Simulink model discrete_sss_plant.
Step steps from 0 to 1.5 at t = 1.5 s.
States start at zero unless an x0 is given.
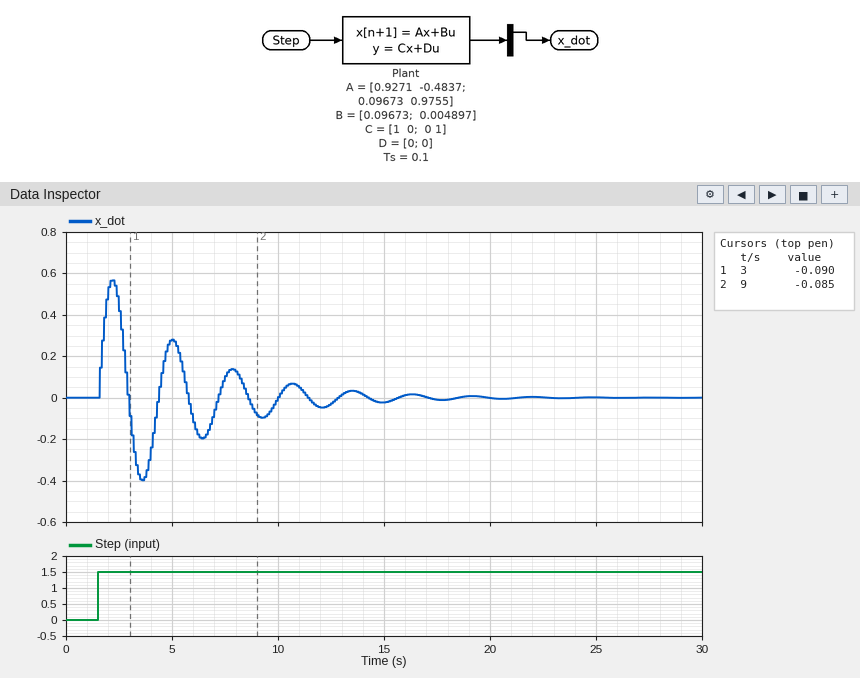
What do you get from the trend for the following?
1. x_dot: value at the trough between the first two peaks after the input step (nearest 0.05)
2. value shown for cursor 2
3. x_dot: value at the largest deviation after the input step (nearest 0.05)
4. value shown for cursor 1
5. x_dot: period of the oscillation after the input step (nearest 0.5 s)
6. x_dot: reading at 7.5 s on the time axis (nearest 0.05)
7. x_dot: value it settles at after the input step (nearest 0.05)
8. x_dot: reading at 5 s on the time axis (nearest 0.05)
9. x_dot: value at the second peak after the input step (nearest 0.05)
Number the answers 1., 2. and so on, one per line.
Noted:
1. -0.40
2. -0.085
3. 0.55
4. -0.090
5. 3.0 s
6. 0.10
7. 0.00
8. 0.30
9. 0.30
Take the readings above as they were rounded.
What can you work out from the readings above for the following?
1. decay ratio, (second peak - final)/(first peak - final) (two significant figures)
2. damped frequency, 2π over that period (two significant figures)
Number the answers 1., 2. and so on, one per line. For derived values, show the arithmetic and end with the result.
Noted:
1. (0.3 - 0) / (0.55 - 0) = 0.55
2. 2π / 3 = 2.1 rad/s
